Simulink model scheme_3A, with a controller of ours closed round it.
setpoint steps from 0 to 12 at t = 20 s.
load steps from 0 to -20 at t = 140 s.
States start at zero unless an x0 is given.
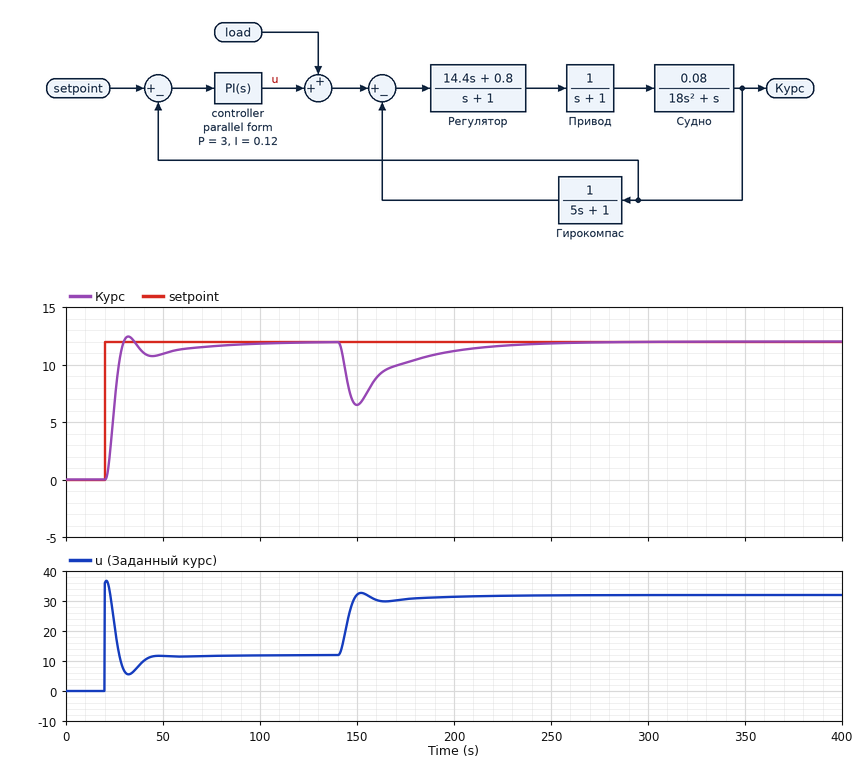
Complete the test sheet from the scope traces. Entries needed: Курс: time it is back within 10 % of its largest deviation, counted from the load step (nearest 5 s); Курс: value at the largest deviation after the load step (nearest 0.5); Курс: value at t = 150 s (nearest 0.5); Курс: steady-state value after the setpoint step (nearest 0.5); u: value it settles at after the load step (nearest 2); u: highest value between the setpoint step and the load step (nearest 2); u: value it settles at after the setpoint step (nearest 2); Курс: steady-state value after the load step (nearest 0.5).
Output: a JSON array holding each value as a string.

["75 s", "6.5", "6.5", "12.0", "32", "36", "12", "12.0"]
